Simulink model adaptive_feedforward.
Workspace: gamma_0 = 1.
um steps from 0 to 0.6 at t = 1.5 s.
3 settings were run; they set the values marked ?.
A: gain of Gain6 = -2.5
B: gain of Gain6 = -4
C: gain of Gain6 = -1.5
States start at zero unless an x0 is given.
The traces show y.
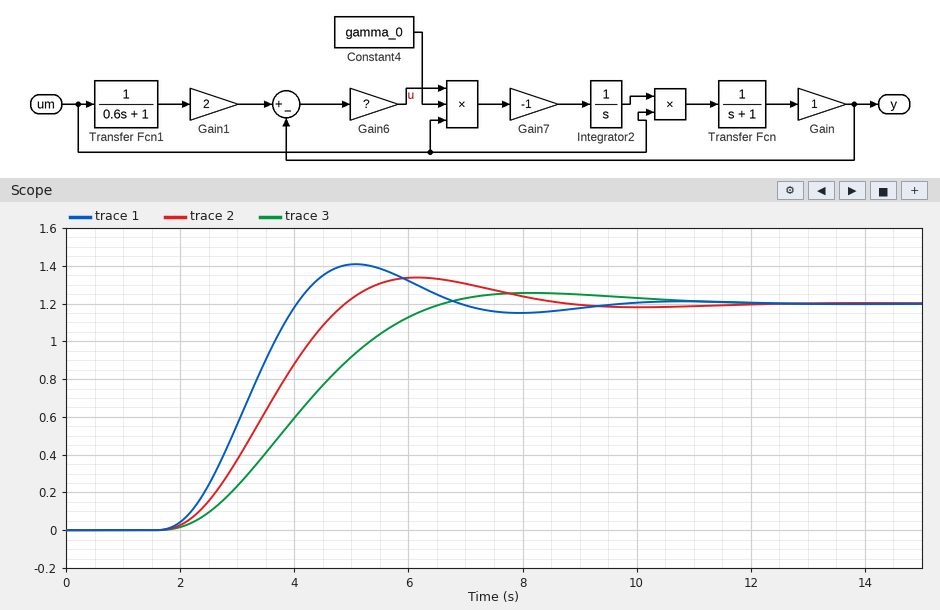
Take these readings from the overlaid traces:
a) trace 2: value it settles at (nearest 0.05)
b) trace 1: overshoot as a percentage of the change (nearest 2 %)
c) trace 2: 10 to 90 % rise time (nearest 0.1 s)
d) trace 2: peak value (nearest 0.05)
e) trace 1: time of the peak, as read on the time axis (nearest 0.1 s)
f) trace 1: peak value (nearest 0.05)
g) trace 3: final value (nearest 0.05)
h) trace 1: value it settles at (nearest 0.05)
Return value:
1.20
18 %
2.1 s
1.35
5.1 s
1.40
1.20
1.20
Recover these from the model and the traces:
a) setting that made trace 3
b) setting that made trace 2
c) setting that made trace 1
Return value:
C
A
B
